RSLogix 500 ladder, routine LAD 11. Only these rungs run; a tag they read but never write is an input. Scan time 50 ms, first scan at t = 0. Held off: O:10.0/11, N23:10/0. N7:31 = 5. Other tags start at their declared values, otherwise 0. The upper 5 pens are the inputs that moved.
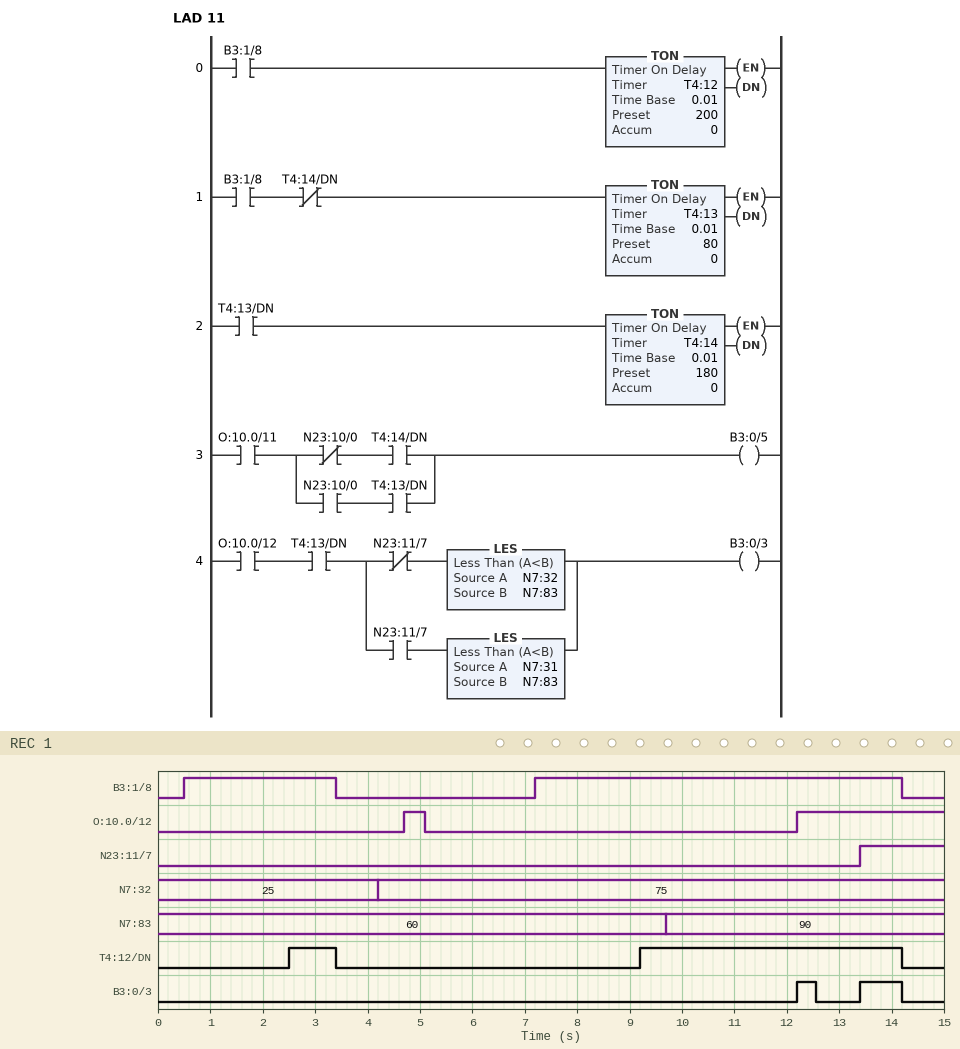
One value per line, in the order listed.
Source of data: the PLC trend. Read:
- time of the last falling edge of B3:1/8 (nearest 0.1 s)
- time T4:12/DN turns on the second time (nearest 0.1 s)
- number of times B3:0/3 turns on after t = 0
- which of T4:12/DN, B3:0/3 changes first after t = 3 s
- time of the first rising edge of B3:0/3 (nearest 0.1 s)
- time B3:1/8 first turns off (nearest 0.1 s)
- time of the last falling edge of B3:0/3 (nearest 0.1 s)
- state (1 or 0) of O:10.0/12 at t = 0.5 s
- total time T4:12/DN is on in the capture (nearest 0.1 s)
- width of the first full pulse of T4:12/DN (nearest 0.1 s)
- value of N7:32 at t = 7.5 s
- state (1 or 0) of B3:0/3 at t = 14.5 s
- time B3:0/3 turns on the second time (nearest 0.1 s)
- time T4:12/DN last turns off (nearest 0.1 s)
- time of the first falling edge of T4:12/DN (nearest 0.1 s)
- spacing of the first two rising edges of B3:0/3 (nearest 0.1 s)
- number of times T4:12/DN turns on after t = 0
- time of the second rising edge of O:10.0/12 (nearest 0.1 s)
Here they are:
14.2 s
9.2 s
2
T4:12/DN
12.2 s
3.4 s
14.2 s
0
5.9 s
0.9 s
75
0
13.4 s
14.2 s
3.4 s
1.2 s
2
12.2 s
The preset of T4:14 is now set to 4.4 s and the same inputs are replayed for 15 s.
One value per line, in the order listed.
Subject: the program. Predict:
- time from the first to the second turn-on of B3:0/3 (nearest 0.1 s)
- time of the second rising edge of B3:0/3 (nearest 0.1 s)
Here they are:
1.1 s
13.3 s
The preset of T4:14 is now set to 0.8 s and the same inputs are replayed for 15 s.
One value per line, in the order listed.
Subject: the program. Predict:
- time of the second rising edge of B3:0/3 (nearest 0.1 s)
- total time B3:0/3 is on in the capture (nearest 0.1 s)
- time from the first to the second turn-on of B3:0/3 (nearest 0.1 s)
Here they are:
13.1 s
0.9 s
0.9 s
